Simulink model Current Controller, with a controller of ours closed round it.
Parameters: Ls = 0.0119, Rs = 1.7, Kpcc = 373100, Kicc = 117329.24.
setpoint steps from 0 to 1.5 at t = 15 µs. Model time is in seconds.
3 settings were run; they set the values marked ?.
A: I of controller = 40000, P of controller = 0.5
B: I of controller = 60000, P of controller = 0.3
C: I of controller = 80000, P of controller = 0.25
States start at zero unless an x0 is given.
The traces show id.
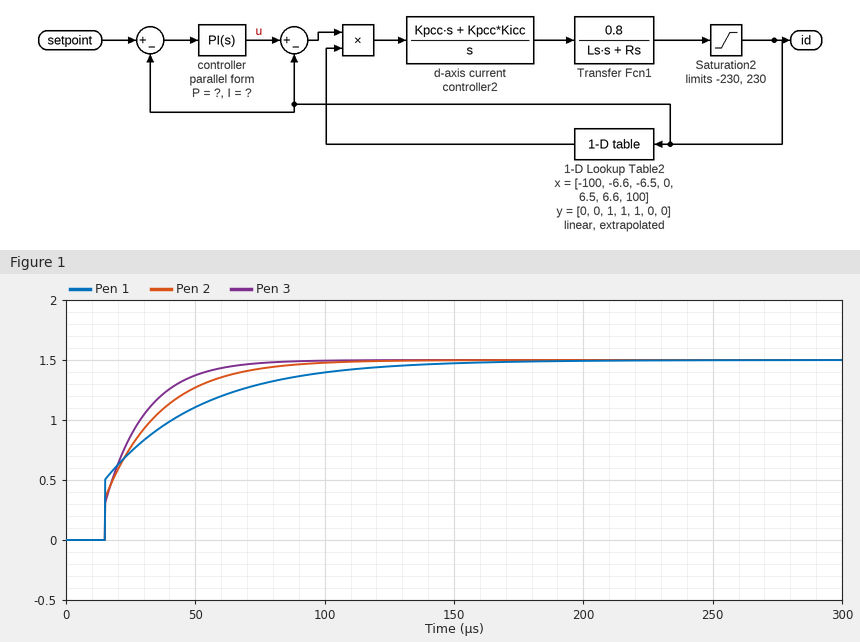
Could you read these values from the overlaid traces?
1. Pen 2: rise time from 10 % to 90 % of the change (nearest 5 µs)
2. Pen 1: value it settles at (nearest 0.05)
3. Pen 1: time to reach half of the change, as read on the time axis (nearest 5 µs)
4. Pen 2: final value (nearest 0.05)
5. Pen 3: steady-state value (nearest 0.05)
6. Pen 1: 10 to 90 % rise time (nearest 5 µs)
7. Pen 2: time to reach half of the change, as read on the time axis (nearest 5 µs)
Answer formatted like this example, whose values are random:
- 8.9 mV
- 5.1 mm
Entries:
- 45 µs
- 1.50
- 25 µs
- 1.50
- 1.50
- 70 µs
- 25 µs
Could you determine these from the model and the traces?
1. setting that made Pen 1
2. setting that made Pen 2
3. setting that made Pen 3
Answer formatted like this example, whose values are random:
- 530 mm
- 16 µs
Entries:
- A
- B
- C
